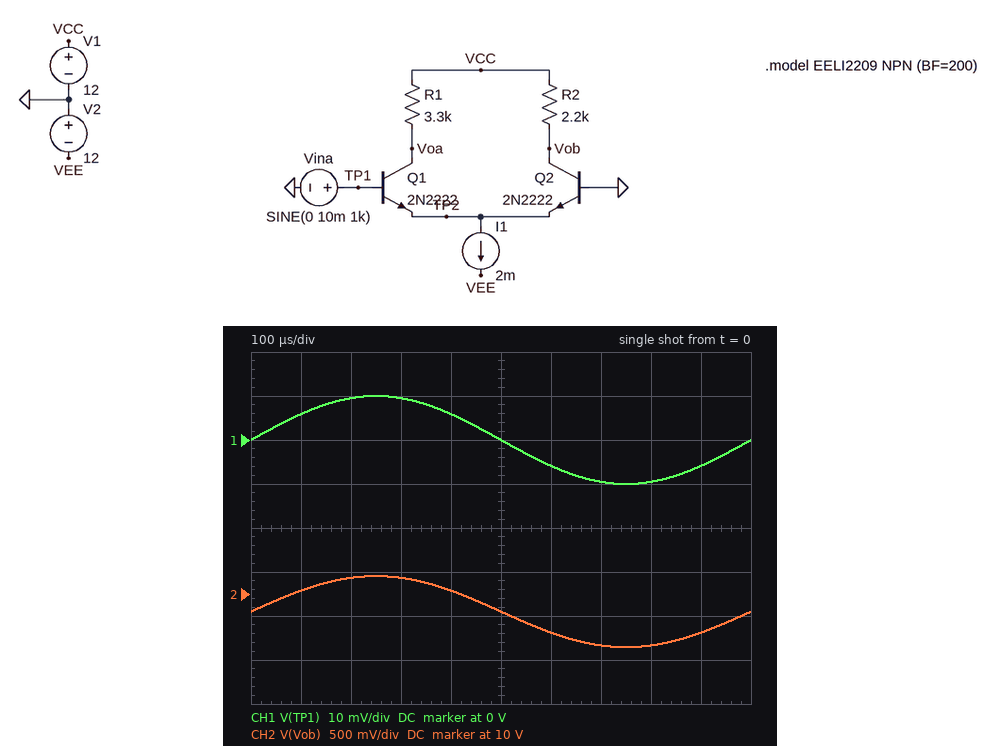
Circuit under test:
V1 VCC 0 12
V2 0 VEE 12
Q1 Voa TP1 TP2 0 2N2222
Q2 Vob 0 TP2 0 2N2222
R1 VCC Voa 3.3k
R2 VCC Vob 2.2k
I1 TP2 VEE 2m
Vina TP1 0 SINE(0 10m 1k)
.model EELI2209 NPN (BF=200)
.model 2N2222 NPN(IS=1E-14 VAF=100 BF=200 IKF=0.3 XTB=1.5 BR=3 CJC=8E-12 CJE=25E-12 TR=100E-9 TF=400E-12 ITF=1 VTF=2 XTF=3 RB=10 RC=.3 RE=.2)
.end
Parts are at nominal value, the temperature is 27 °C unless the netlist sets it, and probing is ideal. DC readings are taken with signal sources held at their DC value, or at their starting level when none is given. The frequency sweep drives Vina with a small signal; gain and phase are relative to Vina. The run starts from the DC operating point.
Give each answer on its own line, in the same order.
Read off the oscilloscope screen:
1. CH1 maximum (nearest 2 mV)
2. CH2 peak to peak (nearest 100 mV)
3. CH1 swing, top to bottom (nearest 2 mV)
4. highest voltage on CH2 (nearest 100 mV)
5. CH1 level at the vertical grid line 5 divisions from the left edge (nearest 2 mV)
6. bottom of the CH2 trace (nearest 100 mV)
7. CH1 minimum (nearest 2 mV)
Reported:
10 mV
800 mV
20 mV
10.2 V
0 V
9.4 V
-10 mV
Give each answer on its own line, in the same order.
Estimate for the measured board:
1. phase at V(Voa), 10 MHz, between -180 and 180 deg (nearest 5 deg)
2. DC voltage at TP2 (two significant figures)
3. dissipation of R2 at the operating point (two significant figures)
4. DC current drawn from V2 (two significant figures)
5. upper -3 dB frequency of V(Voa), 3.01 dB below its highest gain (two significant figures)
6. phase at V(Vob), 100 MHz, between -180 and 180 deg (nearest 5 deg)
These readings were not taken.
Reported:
135 deg
-650 mV
2.2 mW
2.0 mA
11 MHz
-95 deg
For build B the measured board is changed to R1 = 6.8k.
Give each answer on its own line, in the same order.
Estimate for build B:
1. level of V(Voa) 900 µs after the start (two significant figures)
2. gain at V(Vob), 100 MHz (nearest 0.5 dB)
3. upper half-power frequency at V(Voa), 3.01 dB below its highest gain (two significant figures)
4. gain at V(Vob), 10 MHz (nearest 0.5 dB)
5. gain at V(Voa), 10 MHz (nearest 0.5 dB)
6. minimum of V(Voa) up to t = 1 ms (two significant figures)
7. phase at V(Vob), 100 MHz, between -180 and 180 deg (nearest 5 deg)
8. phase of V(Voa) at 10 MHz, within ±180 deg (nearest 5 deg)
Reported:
6.1 V
15.5 dB
4.9 MHz
30.0 dB
34.5 dB
4.1 V
-90 deg
110 deg
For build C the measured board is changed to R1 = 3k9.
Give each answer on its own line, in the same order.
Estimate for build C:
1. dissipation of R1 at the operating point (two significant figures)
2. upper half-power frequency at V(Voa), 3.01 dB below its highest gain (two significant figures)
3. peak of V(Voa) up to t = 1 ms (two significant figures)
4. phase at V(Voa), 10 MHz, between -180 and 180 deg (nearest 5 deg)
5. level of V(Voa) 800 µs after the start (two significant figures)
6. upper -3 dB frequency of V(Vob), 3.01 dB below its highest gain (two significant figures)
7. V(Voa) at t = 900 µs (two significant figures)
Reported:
3.8 mW
9.2 MHz
8.9 V
130 deg
8.8 V
14 MHz
8.6 V
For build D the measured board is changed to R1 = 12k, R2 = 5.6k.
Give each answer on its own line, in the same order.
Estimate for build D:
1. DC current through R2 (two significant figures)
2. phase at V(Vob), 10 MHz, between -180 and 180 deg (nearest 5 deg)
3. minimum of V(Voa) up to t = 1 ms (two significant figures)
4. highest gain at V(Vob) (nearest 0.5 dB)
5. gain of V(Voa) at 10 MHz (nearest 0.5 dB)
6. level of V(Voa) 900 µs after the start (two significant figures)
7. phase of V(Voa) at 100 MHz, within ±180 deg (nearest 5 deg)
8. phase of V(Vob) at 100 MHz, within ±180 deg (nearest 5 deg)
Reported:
1.0 mA
-60 deg
-590 mV
40.0 dB
30.0 dB
1.6 V
60 deg
-100 deg
